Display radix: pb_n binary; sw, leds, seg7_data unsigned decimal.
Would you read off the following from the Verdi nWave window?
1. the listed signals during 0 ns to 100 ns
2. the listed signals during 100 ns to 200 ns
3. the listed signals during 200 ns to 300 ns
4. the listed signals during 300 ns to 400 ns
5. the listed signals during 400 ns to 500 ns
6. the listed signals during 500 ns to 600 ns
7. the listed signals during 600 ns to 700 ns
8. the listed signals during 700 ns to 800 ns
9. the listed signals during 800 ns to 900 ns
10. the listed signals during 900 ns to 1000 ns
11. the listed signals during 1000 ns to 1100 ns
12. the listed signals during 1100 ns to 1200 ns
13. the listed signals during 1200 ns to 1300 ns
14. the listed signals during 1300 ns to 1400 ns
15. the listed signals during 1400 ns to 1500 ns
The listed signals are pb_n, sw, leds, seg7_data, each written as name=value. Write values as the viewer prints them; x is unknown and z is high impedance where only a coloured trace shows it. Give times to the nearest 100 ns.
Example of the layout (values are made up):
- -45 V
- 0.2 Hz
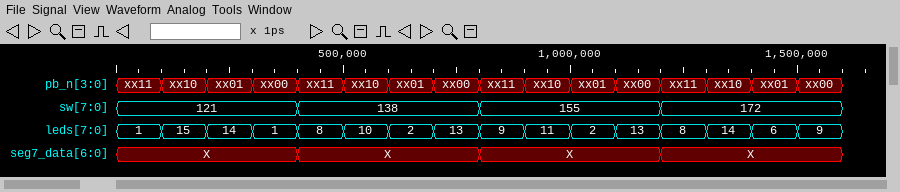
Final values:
- pb_n=xx11, sw=121, leds=1, seg7_data=X
- pb_n=xx10, sw=121, leds=15, seg7_data=X
- pb_n=xx01, sw=121, leds=14, seg7_data=X
- pb_n=xx00, sw=121, leds=1, seg7_data=X
- pb_n=xx11, sw=138, leds=8, seg7_data=X
- pb_n=xx10, sw=138, leds=10, seg7_data=X
- pb_n=xx01, sw=138, leds=2, seg7_data=X
- pb_n=xx00, sw=138, leds=13, seg7_data=X
- pb_n=xx11, sw=155, leds=9, seg7_data=X
- pb_n=xx10, sw=155, leds=11, seg7_data=X
- pb_n=xx01, sw=155, leds=2, seg7_data=X
- pb_n=xx00, sw=155, leds=13, seg7_data=X
- pb_n=xx11, sw=172, leds=8, seg7_data=X
- pb_n=xx10, sw=172, leds=14, seg7_data=X
- pb_n=xx01, sw=172, leds=6, seg7_data=X
